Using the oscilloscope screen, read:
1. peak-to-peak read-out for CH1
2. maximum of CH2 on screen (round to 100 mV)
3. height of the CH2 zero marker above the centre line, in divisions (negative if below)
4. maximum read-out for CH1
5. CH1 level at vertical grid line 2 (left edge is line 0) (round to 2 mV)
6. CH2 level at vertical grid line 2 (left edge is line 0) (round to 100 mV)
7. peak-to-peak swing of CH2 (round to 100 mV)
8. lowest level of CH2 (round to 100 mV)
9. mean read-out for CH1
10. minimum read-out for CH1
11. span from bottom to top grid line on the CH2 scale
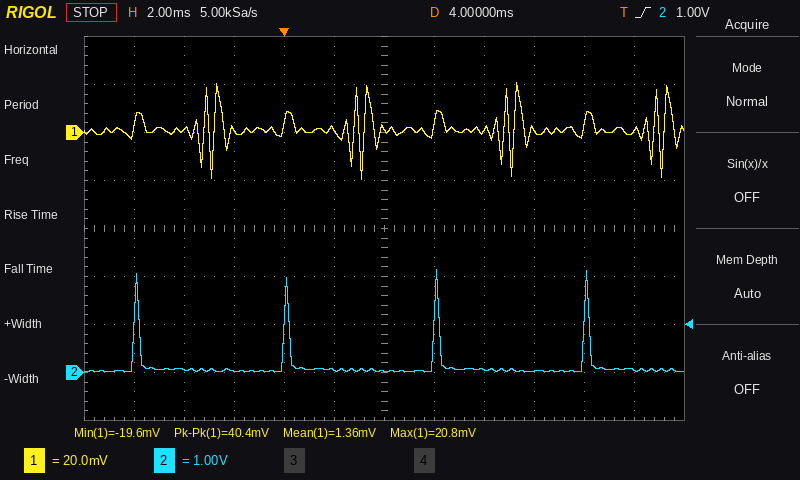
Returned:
40.4 mV
2.1 V
-3.0 div
20.8 mV
2 mV
100 mV
2.1 V
0.0 V
1.36 mV
-19.6 mV
8 V
